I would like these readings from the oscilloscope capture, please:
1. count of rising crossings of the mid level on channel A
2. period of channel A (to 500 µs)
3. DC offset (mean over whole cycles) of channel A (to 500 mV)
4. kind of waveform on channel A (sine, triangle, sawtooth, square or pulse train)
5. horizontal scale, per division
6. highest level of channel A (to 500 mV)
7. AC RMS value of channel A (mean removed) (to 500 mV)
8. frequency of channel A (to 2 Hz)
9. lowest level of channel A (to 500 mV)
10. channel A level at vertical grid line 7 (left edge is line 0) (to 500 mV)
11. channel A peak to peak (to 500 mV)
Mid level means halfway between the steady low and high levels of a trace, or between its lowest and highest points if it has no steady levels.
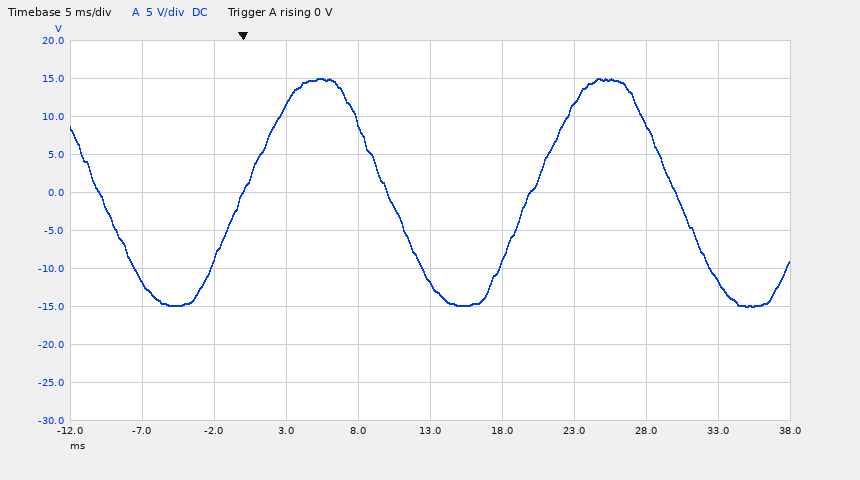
2
20.0 ms
0.0 V
sine
5 ms
15.0 V
10.5 V
50 Hz
-15.0 V
11.5 V
30.0 V
